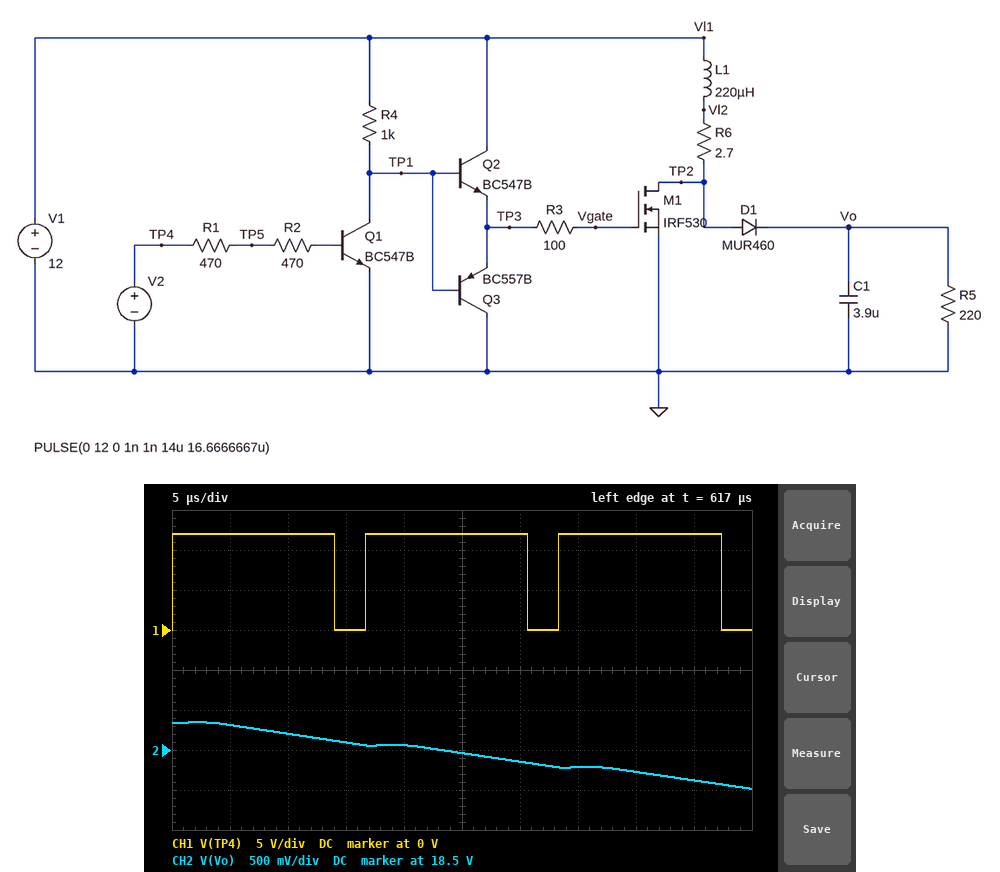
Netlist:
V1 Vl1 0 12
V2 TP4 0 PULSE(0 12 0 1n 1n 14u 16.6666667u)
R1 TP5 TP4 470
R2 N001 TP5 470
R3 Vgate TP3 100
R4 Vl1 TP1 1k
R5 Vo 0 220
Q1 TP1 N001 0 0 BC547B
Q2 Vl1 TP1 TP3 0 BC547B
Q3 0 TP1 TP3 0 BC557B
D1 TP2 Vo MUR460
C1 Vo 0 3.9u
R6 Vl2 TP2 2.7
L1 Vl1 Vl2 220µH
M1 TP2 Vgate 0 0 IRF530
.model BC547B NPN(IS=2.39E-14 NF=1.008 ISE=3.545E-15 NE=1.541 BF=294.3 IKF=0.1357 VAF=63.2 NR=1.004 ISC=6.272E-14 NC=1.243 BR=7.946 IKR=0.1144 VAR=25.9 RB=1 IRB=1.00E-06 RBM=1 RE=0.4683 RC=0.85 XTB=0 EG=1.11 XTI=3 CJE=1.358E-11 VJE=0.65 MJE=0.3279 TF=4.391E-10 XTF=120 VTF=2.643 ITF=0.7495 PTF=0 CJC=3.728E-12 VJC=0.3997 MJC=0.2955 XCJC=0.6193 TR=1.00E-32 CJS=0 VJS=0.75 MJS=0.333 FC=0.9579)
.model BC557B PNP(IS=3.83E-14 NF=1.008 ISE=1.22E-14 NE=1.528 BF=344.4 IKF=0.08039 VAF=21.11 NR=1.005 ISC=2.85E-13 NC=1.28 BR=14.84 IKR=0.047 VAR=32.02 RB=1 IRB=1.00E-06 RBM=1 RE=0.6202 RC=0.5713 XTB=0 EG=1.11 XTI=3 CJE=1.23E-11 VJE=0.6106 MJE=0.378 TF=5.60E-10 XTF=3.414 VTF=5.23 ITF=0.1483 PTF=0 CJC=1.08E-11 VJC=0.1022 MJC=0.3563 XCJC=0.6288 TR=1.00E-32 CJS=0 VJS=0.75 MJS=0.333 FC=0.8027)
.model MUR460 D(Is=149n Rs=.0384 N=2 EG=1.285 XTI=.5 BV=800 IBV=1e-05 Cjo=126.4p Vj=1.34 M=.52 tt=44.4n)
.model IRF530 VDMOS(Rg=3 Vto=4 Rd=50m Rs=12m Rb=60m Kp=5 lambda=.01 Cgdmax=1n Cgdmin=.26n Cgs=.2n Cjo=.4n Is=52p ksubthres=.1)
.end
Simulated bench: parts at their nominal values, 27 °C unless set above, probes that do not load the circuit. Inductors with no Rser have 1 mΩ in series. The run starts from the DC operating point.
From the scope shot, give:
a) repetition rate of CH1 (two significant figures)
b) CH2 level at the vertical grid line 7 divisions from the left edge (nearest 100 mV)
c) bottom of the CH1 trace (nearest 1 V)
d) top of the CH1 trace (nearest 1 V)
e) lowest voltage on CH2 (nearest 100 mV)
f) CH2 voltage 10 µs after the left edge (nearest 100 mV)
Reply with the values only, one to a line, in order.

60 kHz
18.3 V
0 V
12 V
18.0 V
18.7 V
